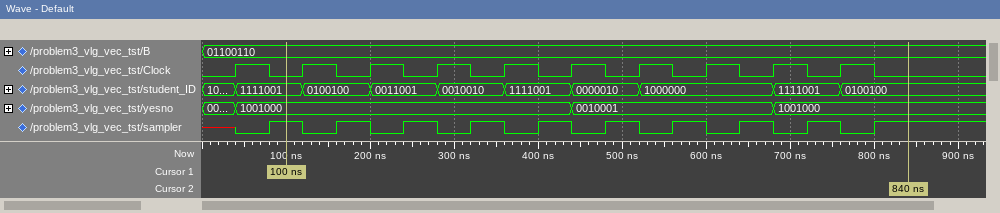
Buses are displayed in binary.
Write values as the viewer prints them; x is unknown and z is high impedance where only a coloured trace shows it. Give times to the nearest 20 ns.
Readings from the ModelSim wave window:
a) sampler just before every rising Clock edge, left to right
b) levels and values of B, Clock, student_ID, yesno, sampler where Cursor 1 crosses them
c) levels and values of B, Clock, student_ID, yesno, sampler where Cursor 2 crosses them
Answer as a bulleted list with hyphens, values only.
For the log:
- x 1 1 1 1 1 1 1 1 1
- B=01100110, Clock=0, student_ID=1111001, yesno=1001000, sampler=1
- B=01100110, Clock=0, student_ID=0100100, yesno=1001000, sampler=1
